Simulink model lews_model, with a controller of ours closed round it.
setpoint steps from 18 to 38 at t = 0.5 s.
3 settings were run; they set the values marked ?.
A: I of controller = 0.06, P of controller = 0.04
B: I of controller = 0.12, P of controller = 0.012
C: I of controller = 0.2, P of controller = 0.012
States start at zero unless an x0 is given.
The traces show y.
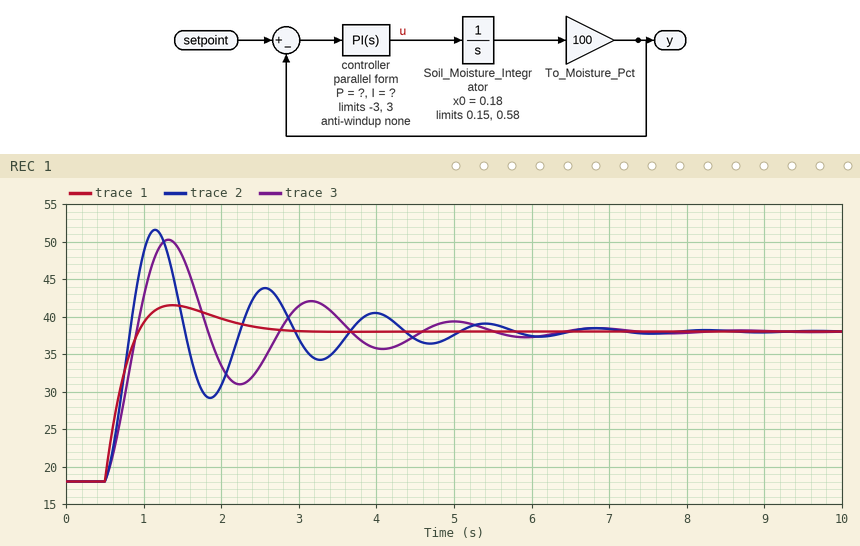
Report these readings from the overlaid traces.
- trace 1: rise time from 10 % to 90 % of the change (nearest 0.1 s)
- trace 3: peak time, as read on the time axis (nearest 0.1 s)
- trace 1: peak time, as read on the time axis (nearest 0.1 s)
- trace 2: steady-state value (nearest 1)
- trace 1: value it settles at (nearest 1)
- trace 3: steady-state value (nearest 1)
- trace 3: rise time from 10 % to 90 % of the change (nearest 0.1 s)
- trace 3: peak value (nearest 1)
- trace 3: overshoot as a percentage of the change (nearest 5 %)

0.3 s
1.3 s
1.4 s
38
38
38
0.3 s
50
60 %
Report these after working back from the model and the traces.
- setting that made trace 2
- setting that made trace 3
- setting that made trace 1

C
B
A
